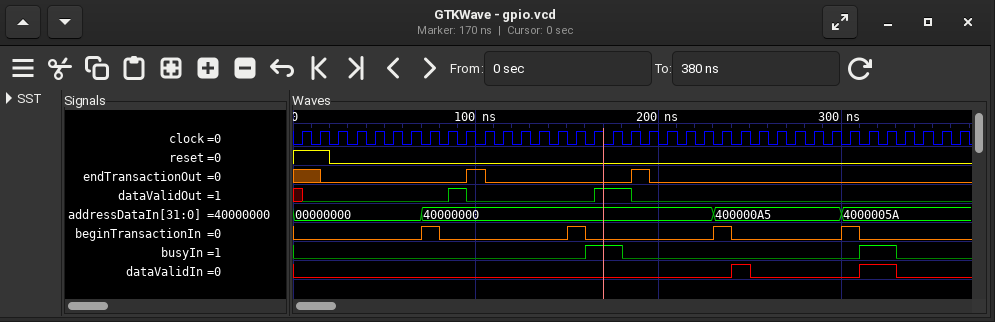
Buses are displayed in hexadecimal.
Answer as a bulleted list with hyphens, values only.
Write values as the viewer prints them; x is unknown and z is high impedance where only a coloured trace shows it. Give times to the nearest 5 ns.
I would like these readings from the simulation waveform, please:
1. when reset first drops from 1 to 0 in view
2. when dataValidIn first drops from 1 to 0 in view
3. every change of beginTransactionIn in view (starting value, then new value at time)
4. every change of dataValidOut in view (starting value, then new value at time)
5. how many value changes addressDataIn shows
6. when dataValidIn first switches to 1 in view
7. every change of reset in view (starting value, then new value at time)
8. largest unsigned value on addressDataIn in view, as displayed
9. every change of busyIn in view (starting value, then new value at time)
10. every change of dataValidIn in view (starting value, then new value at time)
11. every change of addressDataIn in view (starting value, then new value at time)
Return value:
- 20 ns
- 250 ns
- 0, 1 at 70 ns, 0 at 80 ns, 1 at 150 ns, 0 at 160 ns, 1 at 230 ns, 0 at 240 ns, 1 at 300 ns, 0 at 310 ns
- x, 0 at 5 ns, 1 at 85 ns, 0 at 95 ns, 1 at 165 ns, 0 at 185 ns
- 3
- 240 ns
- 1, 0 at 20 ns
- 400000A5
- 0, 1 at 160 ns, 0 at 180 ns, 1 at 310 ns, 0 at 330 ns
- 0, 1 at 240 ns, 0 at 250 ns, 1 at 310 ns, 0 at 330 ns
- 00000000, 40000000 at 70 ns, 400000A5 at 230 ns, 4000005A at 300 ns
